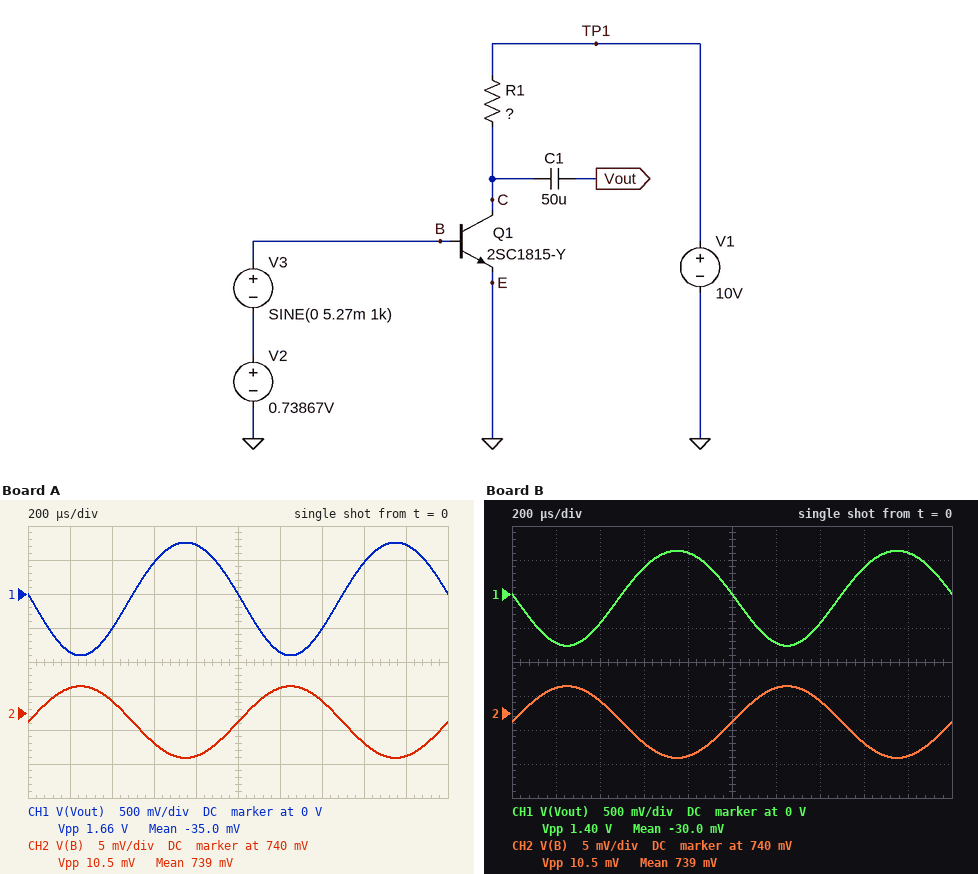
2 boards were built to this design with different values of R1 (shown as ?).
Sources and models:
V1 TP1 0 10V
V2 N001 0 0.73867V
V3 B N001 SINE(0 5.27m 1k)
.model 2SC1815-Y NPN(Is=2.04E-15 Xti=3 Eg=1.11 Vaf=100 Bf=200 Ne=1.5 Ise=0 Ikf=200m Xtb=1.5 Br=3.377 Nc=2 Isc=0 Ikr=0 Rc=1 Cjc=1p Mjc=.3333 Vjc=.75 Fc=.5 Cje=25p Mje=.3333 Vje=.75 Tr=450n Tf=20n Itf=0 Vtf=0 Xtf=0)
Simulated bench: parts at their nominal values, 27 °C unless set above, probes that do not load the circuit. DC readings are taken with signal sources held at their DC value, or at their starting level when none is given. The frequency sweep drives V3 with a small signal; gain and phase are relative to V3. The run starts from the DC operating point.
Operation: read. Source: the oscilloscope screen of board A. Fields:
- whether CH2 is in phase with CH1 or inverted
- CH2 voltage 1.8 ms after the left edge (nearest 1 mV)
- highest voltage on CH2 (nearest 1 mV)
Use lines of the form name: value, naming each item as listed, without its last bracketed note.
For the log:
whether CH2 is in phase with CH1 or inverted: inverted
CH2 voltage 1.8 ms after the left edge: 734 mV
highest voltage on CH2: 744 mV
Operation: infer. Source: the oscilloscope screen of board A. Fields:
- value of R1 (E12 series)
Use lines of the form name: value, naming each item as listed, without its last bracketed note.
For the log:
value of R1: 820 Ω
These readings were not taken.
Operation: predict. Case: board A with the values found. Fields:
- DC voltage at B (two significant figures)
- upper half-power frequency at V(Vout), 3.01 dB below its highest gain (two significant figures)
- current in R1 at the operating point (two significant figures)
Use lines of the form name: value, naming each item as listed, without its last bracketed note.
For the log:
DC voltage at B: 740 mV
upper half-power frequency at V(Vout), 3.01 dB below its highest gain: 400 MHz
current in R1 at the operating point: 5.3 mA
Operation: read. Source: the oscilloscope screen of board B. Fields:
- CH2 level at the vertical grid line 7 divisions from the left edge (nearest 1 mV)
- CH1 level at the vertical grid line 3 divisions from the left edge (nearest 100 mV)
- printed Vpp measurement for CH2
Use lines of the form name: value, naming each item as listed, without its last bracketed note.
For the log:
CH2 level at the vertical grid line 7 divisions from the left edge: 742 mV
CH1 level at the vertical grid line 3 divisions from the left edge: 400 mV
printed Vpp measurement for CH2: 10.5 mV
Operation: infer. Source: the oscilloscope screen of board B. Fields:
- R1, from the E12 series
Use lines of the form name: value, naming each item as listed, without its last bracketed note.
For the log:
R1, from the E12 series: 680 Ω
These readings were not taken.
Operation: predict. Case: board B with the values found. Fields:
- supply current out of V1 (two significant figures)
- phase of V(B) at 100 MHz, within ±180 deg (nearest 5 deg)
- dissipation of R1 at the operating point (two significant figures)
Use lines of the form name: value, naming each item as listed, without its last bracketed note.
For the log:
supply current out of V1: 5.3 mA
phase of V(B) at 100 MHz, within ±180 deg: 0 deg
dissipation of R1 at the operating point: 19 mW
